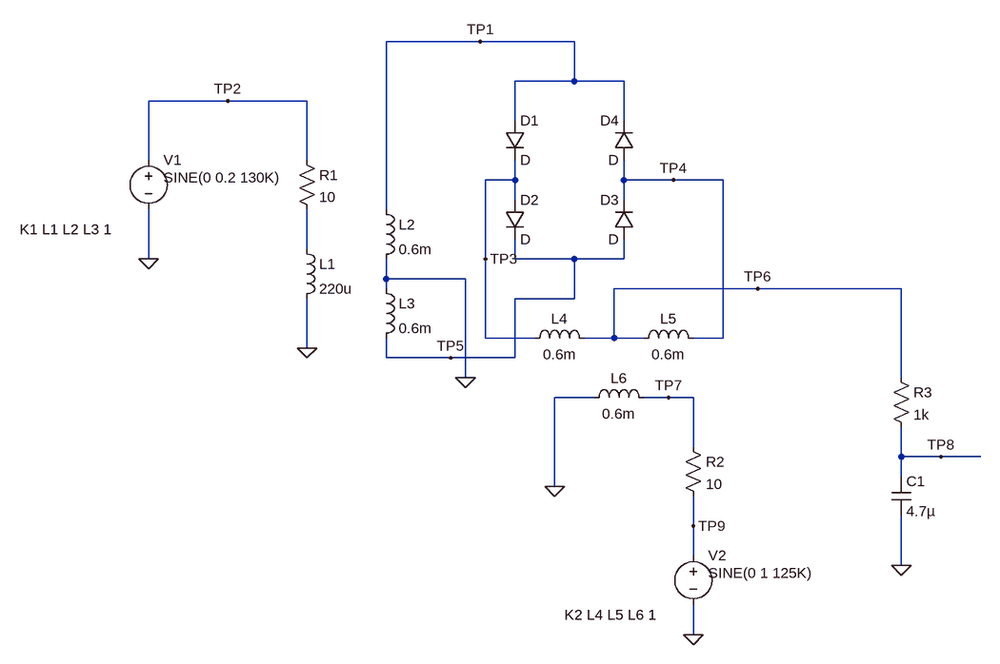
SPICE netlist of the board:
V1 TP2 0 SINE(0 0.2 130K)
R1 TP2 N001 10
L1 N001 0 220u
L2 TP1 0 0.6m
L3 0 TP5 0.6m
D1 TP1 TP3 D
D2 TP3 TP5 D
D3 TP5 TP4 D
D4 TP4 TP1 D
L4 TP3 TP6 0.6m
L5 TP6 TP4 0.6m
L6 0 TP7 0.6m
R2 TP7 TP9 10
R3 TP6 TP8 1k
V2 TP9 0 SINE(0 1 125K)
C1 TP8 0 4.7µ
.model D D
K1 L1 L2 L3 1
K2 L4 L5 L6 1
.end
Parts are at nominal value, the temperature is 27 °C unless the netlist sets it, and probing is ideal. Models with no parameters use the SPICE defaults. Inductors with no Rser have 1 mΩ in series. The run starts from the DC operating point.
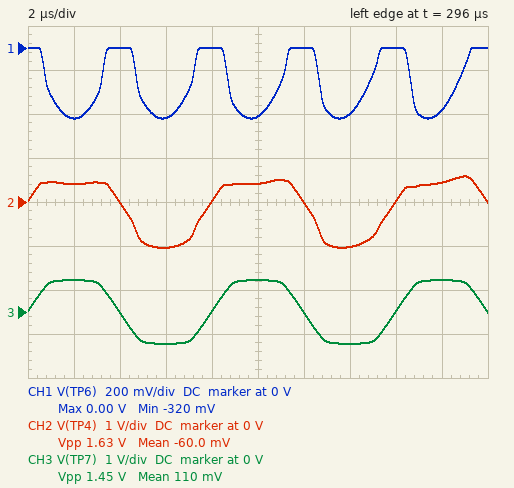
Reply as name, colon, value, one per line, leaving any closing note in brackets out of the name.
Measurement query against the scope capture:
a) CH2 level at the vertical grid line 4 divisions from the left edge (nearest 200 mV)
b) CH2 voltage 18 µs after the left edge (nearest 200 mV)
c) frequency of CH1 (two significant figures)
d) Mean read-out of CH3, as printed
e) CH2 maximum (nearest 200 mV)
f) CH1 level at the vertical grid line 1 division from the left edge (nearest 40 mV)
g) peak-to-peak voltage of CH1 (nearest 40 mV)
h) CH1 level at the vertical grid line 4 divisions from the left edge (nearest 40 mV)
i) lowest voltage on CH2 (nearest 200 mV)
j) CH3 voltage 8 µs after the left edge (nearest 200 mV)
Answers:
CH2 level at the vertical grid line 4 divisions from the left edge: 0 V
CH2 voltage 18 µs after the left edge: 400 mV
frequency of CH1: 260 kHz
Mean read-out of CH3, as printed: 110 mV
CH2 maximum: 600 mV
CH1 level at the vertical grid line 1 division from the left edge: -320 mV
peak-to-peak voltage of CH1: 320 mV
CH1 level at the vertical grid line 4 divisions from the left edge: 0 V
lowest voltage on CH2: -1.0 V
CH3 voltage 8 µs after the left edge: 0 V
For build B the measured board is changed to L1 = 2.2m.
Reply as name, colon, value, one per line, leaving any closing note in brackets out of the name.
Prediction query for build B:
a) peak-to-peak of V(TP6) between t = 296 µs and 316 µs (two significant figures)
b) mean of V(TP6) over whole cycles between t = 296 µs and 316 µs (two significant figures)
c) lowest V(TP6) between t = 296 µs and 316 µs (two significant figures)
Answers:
peak-to-peak of V(TP6) between t = 296 µs and 316 µs: 100 mV
mean of V(TP6) over whole cycles between t = 296 µs and 316 µs: -55 mV
lowest V(TP6) between t = 296 µs and 316 µs: -100 mV
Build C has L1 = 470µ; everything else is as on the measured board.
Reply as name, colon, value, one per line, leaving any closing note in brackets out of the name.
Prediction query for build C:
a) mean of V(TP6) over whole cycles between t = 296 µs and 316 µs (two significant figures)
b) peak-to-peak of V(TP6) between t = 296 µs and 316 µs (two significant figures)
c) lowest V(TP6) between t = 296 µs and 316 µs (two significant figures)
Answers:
mean of V(TP6) over whole cycles between t = 296 µs and 316 µs: -120 mV
peak-to-peak of V(TP6) between t = 296 µs and 316 µs: 220 mV
lowest V(TP6) between t = 296 µs and 316 µs: -220 mV
